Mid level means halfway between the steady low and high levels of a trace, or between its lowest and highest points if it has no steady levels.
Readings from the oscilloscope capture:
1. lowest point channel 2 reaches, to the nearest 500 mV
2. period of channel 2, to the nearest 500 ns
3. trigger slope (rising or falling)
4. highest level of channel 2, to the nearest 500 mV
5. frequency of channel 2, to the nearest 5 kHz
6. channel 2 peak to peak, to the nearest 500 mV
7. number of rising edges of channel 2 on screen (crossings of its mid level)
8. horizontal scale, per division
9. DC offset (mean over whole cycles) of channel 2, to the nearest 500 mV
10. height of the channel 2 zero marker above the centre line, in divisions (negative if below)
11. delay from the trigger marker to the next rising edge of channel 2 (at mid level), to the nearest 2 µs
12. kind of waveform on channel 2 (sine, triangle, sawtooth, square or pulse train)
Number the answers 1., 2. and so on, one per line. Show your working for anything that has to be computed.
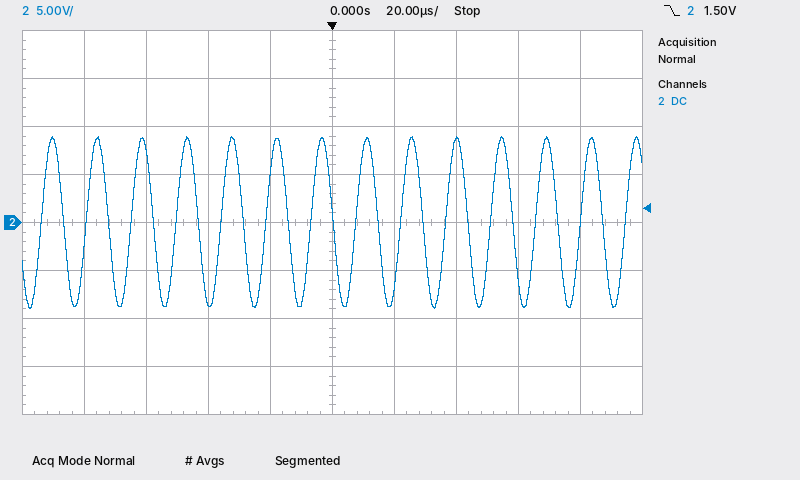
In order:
1. -9.0 V
2. 14.5 µs
3. falling
4. 9.0 V
5. 1 / 14.5 µs ≈ 69.0 kHz, so 70 kHz to the nearest 5 kHz
6. 9.0 V − (-9.0 V) = 18.0 V
7. 14
8. 20 µs
9. (9.0 V + (-9.0 V)) / 2 ≈ 0.0 V
10. 0.0 div
11. 8 µs
12. sine
